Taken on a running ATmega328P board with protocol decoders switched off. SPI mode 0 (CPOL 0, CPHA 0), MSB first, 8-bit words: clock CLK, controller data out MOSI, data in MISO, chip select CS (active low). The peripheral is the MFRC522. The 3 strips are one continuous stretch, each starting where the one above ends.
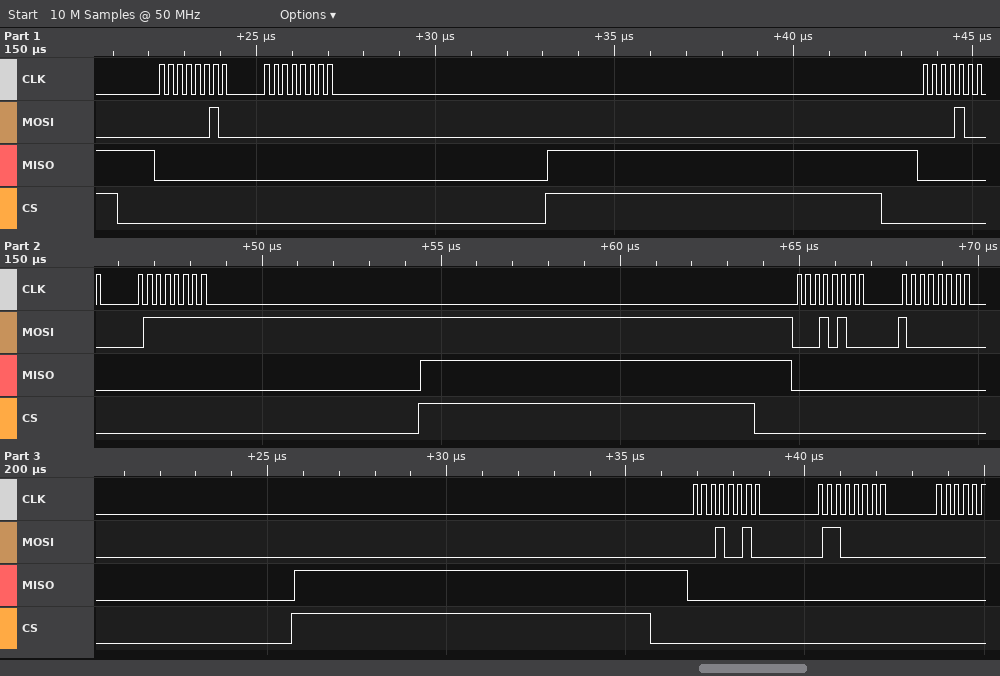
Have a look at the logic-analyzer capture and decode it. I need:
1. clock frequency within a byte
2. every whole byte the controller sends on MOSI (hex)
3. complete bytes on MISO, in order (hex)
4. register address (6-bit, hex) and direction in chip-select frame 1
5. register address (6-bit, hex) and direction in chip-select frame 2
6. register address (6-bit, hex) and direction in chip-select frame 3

4 MHz
02 00 08 7F 14 80 12 60
00 00 00 00 00 00 00 00
0x01 write
0x04 write
0x0A write
